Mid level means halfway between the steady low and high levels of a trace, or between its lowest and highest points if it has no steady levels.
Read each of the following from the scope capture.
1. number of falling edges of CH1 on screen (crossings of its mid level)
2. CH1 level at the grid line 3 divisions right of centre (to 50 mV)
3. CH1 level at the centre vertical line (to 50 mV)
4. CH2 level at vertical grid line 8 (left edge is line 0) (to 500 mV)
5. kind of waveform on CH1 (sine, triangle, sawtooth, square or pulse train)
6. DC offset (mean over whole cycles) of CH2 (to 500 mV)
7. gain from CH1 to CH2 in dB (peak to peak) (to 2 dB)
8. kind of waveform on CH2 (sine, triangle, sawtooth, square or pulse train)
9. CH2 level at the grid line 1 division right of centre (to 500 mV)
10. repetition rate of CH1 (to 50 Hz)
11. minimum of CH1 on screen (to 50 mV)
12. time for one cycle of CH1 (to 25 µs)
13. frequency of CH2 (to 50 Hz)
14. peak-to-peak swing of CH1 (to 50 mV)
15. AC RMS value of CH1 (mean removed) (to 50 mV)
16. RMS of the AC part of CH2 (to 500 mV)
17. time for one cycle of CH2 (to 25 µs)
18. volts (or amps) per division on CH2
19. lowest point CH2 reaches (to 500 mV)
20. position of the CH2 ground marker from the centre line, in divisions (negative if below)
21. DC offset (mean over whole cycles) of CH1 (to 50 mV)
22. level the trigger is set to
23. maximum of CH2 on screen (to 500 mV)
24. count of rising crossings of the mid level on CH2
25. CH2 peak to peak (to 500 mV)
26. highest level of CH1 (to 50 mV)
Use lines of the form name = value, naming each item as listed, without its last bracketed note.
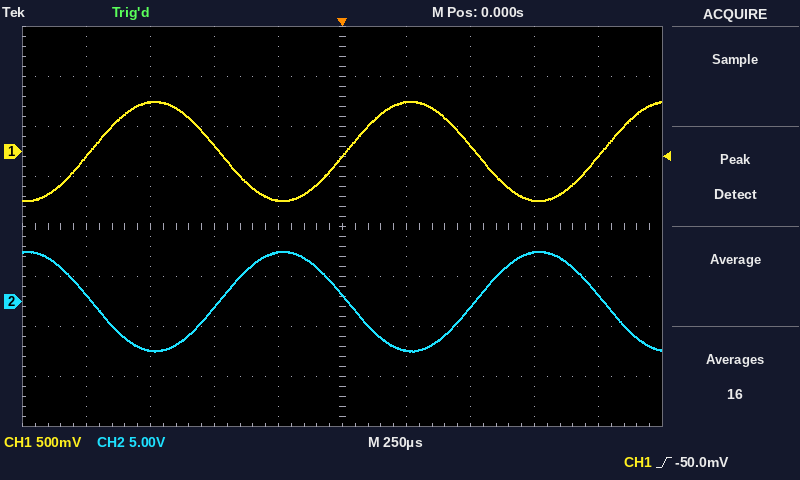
number of falling edges of CH1 on screen = 2
CH1 level at the grid line 3 divisions right of centre = -500 mV
CH1 level at the centre vertical line = -50 mV
CH2 level at vertical grid line 8 (left edge is line 0) = 5.0 V
kind of waveform on CH1 = sine
DC offset (mean over whole cycles) of CH2 = 0.0 V
gain from CH1 to CH2 in dB (peak to peak) = 20 dB
kind of waveform on CH2 = sine
CH2 level at the grid line 1 division right of centre = -5.0 V
repetition rate of CH1 = 1.00 kHz
minimum of CH1 on screen = -500 mV
time for one cycle of CH1 = 1.000 ms
frequency of CH2 = 1.00 kHz
peak-to-peak swing of CH1 = 1.00 V
AC RMS value of CH1 (mean removed) = 350 mV
RMS of the AC part of CH2 = 3.5 V
time for one cycle of CH2 = 1.000 ms
volts (or amps) per division on CH2 = 5 V
lowest point CH2 reaches = -5.0 V
position of the CH2 ground marker from the centre line, in divisions = -1.5 div
DC offset (mean over whole cycles) of CH1 = 0 mV
level the trigger is set to = -50.0 mV
maximum of CH2 on screen = 5.0 V
count of rising crossings of the mid level on CH2 = 2
CH2 peak to peak = 10.0 V
highest level of CH1 = 500 mV
